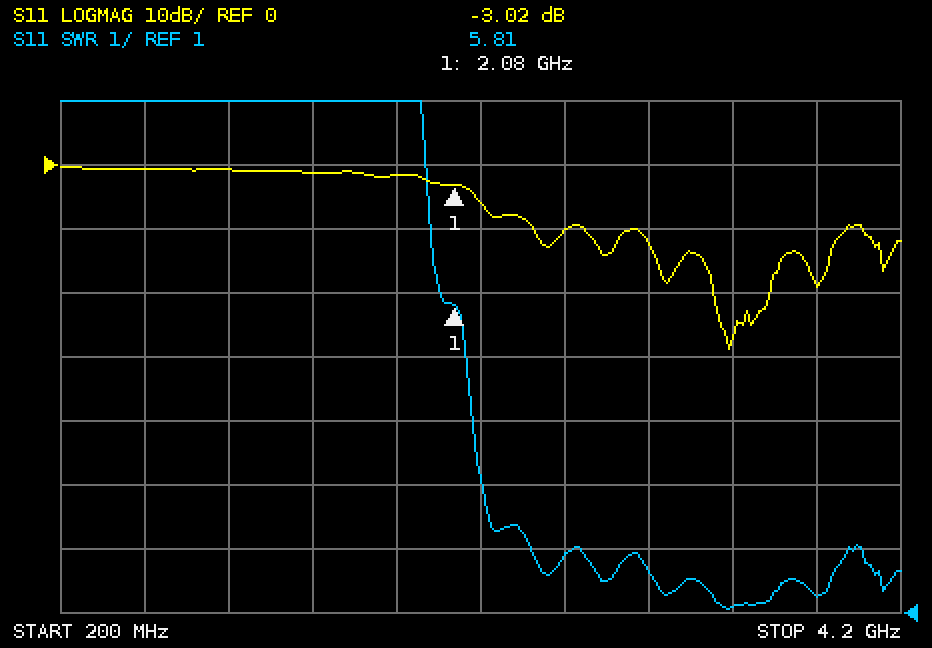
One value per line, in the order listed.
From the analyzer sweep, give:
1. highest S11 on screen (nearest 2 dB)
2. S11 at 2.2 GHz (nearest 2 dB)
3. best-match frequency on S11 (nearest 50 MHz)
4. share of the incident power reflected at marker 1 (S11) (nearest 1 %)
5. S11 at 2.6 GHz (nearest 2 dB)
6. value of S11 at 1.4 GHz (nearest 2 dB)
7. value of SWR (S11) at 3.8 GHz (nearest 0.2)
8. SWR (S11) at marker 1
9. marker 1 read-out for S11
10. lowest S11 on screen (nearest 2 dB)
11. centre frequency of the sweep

0 dB
-6 dB
3.40 GHz
50 %
-10 dB
-2 dB
1.2
5.81
-3.02 dB
-28 dB
2.2 GHz
